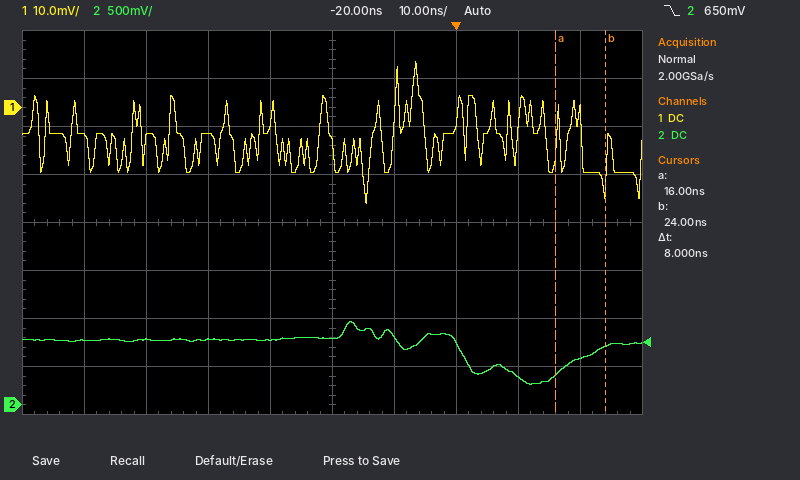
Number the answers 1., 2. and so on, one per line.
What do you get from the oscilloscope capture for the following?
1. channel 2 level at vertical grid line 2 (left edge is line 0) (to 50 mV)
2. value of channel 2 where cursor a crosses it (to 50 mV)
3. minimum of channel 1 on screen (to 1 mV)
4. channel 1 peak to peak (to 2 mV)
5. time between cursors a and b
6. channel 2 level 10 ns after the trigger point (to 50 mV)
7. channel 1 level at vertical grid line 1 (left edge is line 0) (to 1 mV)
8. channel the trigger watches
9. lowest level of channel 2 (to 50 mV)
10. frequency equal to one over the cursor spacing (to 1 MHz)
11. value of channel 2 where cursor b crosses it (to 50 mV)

1. 700 mV
2. 300 mV
3. -20 mV
4. 30 mV
5. 8 ns
6. 300 mV
7. -6 mV
8. channel 2
9. 200 mV
10. 125 MHz
11. 600 mV
